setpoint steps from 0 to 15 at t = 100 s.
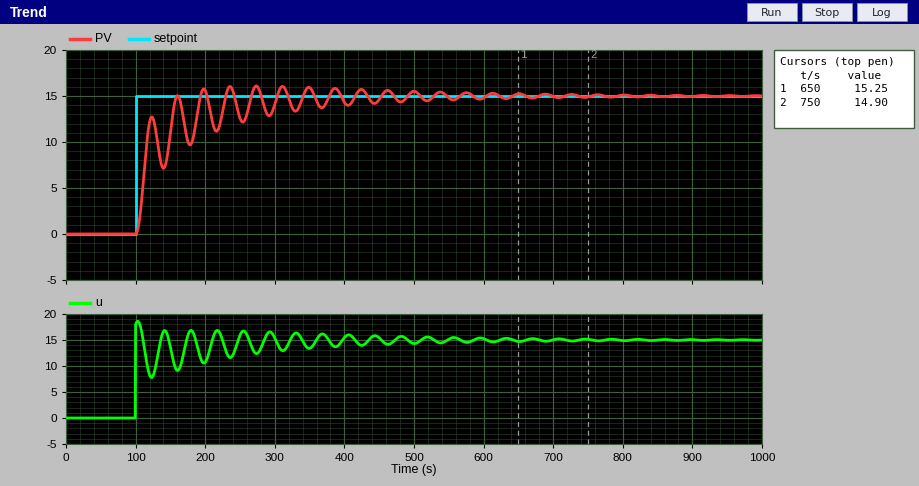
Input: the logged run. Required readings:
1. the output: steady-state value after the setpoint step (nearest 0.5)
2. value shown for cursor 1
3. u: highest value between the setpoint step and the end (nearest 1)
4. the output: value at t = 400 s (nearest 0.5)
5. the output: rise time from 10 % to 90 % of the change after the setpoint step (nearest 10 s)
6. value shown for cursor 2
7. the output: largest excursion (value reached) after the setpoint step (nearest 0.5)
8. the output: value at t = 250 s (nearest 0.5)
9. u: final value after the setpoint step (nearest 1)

15.0
15.25
19
14.5
50 s
14.90
16.0
12.5
15
